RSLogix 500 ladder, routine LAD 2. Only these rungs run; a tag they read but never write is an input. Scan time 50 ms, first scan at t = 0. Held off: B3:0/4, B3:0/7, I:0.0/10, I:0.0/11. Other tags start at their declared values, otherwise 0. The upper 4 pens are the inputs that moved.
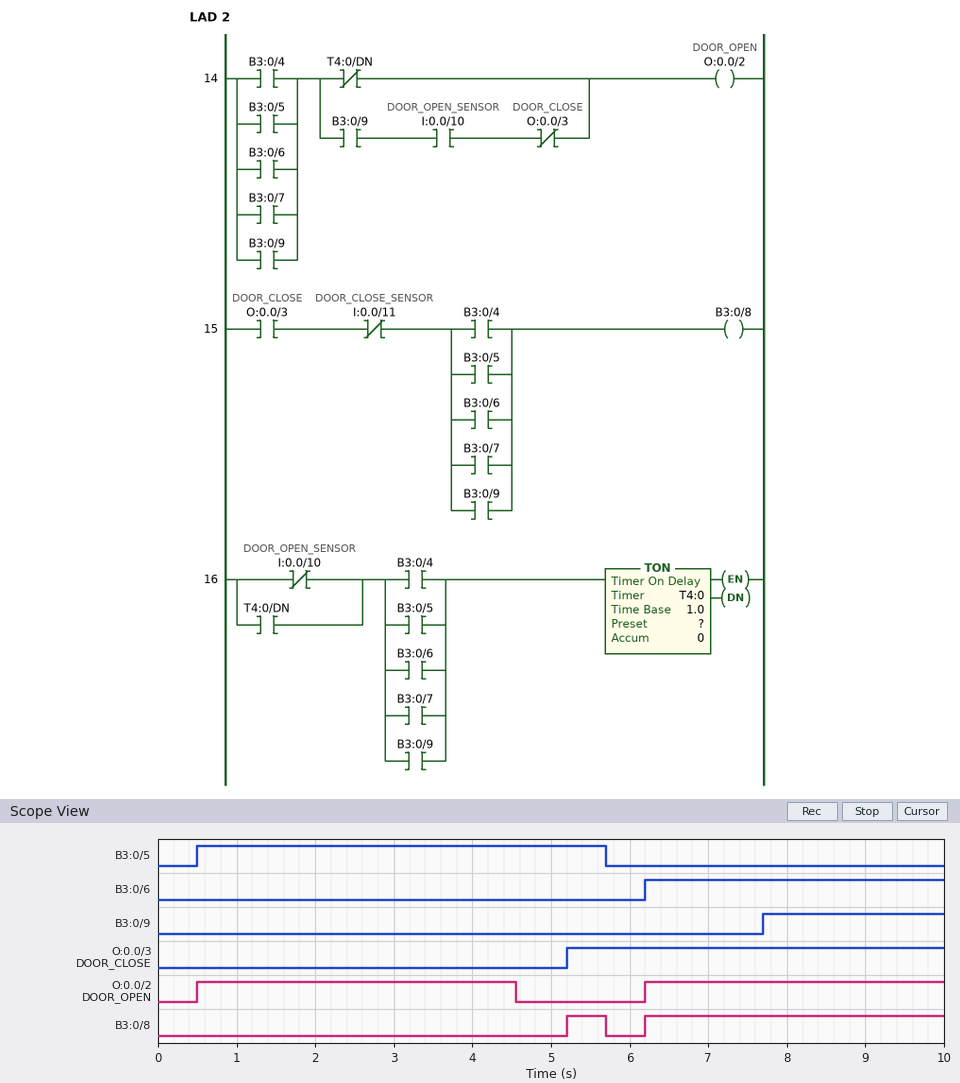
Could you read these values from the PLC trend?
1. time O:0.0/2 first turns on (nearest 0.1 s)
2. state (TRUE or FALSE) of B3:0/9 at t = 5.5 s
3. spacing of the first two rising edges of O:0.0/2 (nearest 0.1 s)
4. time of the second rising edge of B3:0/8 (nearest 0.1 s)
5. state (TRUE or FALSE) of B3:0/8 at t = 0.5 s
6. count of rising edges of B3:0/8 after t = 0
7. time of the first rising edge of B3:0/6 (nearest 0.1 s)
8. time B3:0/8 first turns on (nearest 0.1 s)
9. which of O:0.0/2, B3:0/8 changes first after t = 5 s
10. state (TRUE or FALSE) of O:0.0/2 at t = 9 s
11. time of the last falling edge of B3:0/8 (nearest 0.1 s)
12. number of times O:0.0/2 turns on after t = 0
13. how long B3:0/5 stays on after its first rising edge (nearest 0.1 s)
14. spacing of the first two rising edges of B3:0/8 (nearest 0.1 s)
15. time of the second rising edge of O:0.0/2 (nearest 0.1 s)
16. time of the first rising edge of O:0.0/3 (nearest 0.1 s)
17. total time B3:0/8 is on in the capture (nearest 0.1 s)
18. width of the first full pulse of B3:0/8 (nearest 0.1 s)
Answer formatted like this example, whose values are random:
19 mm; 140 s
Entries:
0.5 s; FALSE; 5.7 s; 6.2 s; FALSE; 2; 6.2 s; 5.2 s; B3:0/8; TRUE; 5.7 s; 2; 5.2 s; 1.0 s; 6.2 s; 5.2 s; 4.3 s; 0.5 s
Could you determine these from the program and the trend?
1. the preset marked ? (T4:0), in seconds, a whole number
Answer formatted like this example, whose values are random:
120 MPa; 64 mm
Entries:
4 s
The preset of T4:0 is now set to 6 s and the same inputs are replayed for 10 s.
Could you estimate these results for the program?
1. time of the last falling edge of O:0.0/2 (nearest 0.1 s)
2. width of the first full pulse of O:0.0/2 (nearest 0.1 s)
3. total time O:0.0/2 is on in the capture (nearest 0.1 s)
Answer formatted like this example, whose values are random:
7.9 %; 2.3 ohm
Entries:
5.7 s; 5.2 s; 9.0 s
